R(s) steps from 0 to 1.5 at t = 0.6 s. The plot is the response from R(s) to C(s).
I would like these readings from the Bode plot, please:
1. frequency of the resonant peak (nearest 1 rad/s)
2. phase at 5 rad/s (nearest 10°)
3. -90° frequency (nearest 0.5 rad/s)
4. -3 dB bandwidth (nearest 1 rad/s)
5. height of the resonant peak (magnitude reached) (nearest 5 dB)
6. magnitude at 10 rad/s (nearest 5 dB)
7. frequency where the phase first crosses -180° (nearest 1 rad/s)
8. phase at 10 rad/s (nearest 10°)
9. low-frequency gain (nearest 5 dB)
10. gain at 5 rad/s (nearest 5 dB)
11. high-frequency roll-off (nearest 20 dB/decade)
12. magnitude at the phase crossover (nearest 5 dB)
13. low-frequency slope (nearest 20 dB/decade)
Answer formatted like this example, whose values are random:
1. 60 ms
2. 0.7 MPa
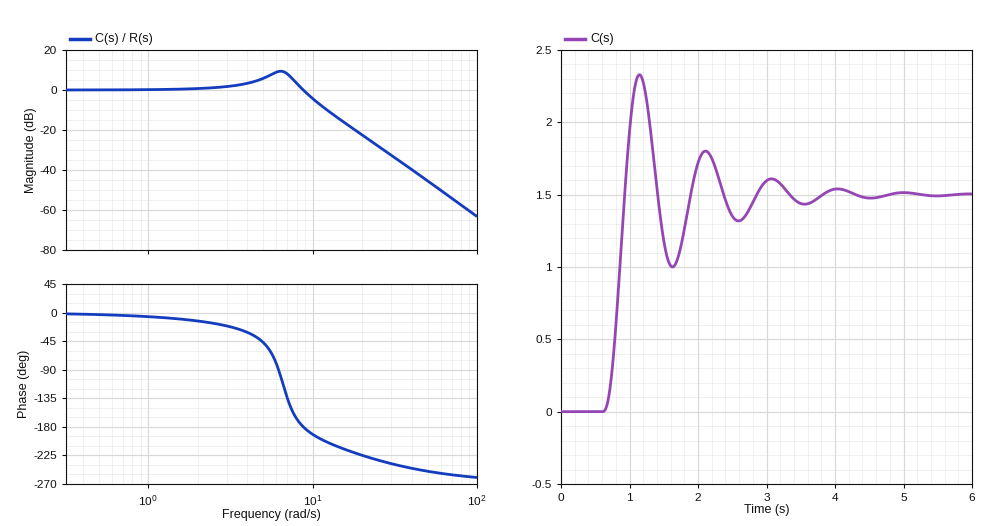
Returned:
1. 6 rad/s
2. -50°
3. 6.0 rad/s
4. 10 rad/s
5. 10 dB
6. -5 dB
7. 9 rad/s
8. -190°
9. 0 dB
10. 5 dB
11. -60 dB/decade
12. 0 dB
13. 0 dB/decade
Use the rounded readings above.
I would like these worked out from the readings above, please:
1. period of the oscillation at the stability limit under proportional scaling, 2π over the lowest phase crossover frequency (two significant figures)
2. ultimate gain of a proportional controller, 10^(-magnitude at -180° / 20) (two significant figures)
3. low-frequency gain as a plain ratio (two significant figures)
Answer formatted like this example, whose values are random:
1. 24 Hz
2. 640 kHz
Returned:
1. 0.70 s
2. 1.0
3. 1.0
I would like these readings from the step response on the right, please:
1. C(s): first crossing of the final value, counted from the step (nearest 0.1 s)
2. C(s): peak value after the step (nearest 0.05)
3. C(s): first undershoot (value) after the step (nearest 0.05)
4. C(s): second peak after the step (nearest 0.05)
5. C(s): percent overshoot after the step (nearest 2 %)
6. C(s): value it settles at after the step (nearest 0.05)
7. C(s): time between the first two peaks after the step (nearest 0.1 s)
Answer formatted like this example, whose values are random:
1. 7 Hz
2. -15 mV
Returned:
1. 0.3 s
2. 2.35
3. 1.00
4. 1.80
5. 56 %
6. 1.50
7. 1.0 s
